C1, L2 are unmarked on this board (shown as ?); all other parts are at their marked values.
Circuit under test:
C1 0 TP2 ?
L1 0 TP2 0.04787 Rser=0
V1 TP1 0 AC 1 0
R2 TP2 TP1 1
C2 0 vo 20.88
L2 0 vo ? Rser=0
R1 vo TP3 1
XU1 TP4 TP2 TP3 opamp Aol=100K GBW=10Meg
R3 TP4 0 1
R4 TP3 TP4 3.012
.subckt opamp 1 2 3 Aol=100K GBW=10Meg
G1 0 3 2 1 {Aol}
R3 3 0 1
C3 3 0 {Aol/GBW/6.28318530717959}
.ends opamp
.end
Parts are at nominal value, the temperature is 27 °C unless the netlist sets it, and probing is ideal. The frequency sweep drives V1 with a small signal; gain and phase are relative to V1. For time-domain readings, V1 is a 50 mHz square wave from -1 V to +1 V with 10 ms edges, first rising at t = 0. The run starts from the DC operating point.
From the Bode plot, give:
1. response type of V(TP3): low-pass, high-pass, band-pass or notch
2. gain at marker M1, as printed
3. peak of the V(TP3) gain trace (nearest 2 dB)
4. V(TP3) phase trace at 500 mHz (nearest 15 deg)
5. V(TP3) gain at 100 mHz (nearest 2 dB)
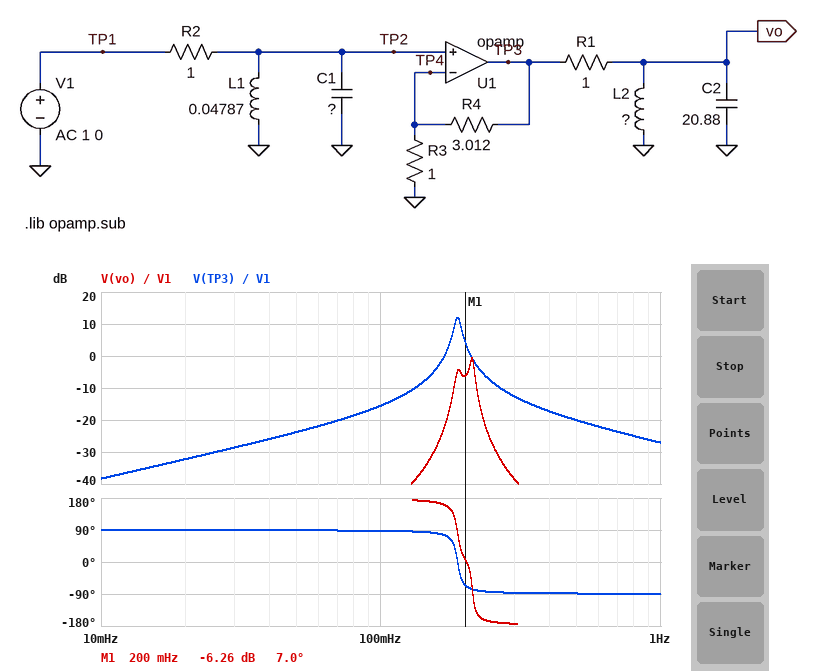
band-pass
-6.26 dB
12 dB
-90 deg
-16 dB
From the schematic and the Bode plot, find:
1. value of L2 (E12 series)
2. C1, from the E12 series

27 mH
15 F
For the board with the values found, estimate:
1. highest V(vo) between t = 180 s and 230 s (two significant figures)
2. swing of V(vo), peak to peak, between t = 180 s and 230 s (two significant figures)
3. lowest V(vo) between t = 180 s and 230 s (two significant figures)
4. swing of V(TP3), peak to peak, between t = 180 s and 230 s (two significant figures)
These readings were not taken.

22 mV
44 mV
-22 mV
550 mV
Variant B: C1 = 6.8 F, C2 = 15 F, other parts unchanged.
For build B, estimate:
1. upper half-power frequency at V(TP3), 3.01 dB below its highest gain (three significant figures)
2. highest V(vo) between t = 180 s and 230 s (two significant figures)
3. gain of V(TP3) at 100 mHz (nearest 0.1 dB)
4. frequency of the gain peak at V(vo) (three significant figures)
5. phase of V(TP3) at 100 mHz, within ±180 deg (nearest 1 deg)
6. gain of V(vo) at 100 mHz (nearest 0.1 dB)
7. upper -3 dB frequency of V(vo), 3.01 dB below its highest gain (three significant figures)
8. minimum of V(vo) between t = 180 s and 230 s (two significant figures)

291 mHz
370 mV
-17.2 dB
251 mHz
88 deg
-51.1 dB
259 mHz
-370 mV
